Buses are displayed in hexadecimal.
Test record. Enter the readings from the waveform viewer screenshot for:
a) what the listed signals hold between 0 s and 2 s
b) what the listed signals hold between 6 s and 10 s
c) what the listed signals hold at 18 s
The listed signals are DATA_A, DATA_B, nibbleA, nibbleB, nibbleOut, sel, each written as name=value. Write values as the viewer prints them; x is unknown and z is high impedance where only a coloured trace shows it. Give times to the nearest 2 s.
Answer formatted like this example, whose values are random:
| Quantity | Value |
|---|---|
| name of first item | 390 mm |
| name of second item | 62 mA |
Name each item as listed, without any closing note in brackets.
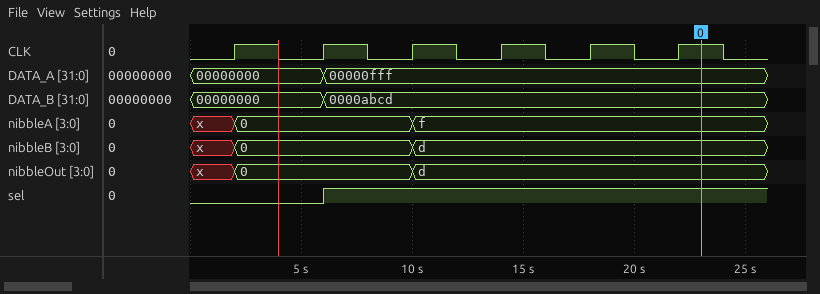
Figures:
| Quantity | Value |
|---|---|
| what the listed signals hold between 0 s and 2 s | DATA_A=00000000, DATA_B=00000000, nibbleA=x, nibbleB=x, nibbleOut=x, sel=0 |
| what the listed signals hold between 6 s and 10 s | DATA_A=00000fff, DATA_B=0000abcd, nibbleA=0, nibbleB=0, nibbleOut=0, sel=1 |
| what the listed signals hold at 18 s | DATA_A=00000fff, DATA_B=0000abcd, nibbleA=f, nibbleB=d, nibbleOut=d, sel=1 |
